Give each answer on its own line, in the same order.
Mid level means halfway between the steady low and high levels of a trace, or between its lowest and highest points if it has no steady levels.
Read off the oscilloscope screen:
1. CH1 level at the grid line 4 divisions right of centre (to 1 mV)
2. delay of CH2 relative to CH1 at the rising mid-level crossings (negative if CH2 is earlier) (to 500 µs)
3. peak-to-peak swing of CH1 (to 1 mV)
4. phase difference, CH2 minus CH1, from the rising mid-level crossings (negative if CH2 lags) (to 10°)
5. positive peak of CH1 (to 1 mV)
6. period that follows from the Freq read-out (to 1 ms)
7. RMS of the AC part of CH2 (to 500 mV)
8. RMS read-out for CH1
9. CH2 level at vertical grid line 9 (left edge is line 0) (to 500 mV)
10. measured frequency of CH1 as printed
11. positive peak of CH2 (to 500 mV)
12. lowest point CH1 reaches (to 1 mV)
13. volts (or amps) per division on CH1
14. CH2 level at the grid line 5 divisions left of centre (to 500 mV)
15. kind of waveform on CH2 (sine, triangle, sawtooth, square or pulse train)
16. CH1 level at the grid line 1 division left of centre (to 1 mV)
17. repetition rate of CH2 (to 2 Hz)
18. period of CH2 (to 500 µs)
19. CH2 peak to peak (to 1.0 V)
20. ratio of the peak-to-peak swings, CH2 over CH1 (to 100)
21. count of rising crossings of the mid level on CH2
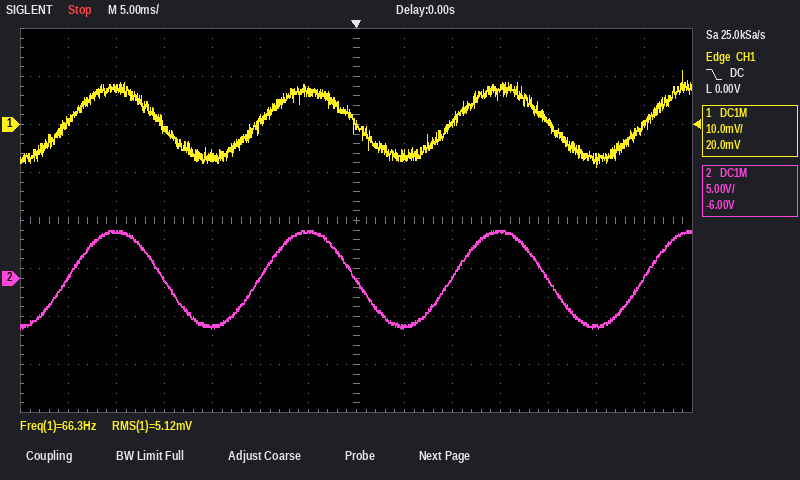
1 mV
-500 µs
20 mV
+10°
11 mV
15 ms
3.5 V
5.12 mV
0.0 V
66.3 Hz
5.0 V
-9 mV
10 mV
5.0 V
sine
7 mV
50 Hz
20.0 ms
10.0 V
500
4
